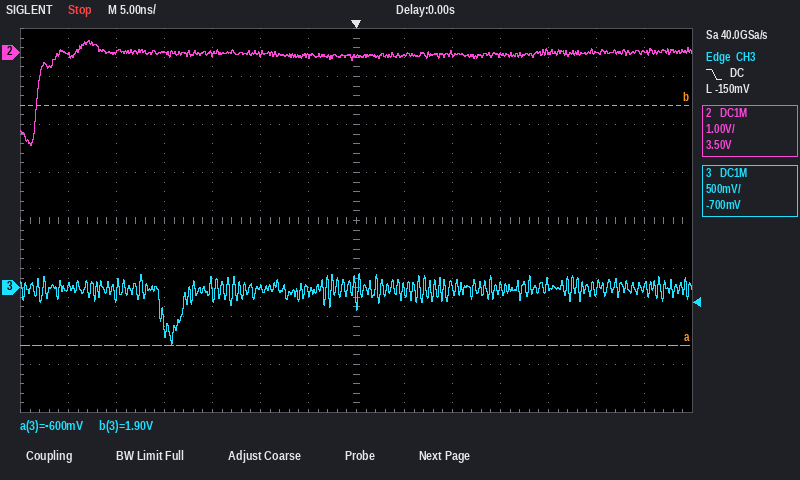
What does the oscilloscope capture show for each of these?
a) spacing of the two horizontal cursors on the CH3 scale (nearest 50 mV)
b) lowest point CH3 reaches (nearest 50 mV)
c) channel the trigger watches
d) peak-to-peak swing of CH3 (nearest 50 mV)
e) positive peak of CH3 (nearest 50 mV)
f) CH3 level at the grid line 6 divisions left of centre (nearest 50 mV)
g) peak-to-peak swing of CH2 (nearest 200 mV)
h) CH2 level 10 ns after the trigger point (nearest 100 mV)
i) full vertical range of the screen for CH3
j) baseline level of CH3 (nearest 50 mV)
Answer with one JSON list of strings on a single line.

["2.50 V", "-600 mV", "CH3", "750 mV", "150 mV", "0 mV", "2.2 V", "0.0 V", "4 V", "0 mV"]
